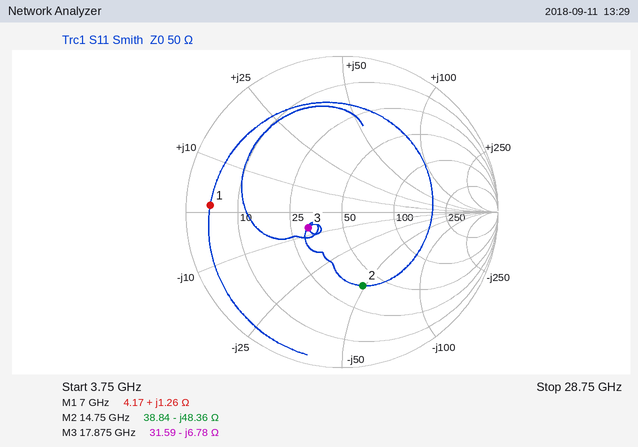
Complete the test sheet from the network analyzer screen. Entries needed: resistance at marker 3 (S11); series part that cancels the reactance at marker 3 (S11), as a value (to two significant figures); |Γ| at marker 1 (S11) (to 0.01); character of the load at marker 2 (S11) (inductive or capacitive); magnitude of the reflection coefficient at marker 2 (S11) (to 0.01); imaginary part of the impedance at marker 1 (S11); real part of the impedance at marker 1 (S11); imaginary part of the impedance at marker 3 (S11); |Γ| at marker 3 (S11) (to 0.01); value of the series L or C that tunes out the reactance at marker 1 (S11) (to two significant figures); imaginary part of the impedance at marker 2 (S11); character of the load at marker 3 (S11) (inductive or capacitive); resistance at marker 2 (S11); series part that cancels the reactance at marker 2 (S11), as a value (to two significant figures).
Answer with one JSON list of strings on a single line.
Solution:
["31.59 Ω", "60 pH", "0.85", "capacitive", "0.49", "+1.26 Ω", "4.17 Ω", "-6.78 Ω", "0.24", "18 pF", "-48.36 Ω", "capacitive", "38.84 Ω", "520 pH"]
